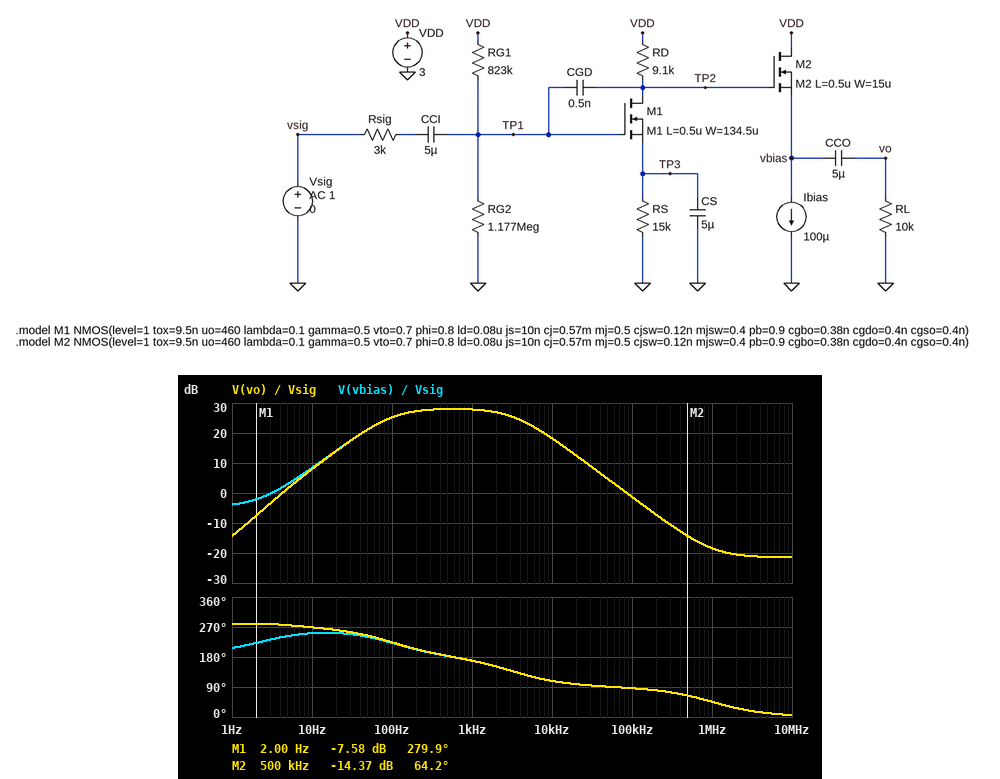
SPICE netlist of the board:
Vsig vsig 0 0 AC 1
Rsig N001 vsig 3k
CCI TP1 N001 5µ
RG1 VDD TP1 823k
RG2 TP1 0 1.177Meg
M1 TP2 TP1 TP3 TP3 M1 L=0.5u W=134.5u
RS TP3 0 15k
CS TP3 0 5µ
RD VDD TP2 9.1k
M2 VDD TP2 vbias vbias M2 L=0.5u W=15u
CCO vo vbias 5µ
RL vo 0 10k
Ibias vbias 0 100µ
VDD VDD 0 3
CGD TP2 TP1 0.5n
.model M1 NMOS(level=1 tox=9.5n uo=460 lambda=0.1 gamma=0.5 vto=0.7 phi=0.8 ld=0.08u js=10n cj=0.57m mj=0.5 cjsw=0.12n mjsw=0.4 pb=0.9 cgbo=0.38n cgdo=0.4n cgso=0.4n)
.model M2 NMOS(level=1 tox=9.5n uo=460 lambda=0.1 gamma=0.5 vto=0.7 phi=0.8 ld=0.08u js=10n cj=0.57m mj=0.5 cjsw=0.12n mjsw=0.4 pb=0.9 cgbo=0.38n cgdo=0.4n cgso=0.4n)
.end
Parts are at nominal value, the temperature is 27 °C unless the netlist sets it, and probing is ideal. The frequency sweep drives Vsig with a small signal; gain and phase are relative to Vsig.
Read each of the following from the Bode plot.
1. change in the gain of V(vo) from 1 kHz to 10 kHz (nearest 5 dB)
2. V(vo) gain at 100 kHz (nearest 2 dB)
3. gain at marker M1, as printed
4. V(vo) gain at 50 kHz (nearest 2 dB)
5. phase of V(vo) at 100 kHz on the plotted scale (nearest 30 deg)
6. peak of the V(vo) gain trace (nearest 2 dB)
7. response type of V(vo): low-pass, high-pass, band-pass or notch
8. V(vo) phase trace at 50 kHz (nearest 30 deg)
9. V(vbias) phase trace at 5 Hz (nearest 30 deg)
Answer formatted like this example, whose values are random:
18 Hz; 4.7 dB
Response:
-10 dB; -2 dB; -7.58 dB; 4 dB; 90 deg; 28 dB; band-pass; 90 deg; 240 deg
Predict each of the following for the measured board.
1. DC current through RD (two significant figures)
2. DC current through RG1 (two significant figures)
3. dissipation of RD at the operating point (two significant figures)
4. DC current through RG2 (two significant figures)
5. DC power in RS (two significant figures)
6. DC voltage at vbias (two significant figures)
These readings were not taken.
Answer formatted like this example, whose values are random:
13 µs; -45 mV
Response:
68 µA; 1.5 µA; 42 µW; 1.5 µA; 70 µW; 1.5 V
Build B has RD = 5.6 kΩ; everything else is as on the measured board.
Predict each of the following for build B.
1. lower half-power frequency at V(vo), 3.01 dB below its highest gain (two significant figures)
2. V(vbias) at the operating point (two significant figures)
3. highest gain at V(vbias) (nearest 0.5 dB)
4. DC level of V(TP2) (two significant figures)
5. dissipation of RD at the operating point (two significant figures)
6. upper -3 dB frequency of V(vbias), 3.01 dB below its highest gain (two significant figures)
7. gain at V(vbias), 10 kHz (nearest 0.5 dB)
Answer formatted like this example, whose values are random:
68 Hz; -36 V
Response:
100 Hz; 1.8 V; 24.0 dB; 2.6 V; 26 µW; 5.4 kHz; 17.5 dB
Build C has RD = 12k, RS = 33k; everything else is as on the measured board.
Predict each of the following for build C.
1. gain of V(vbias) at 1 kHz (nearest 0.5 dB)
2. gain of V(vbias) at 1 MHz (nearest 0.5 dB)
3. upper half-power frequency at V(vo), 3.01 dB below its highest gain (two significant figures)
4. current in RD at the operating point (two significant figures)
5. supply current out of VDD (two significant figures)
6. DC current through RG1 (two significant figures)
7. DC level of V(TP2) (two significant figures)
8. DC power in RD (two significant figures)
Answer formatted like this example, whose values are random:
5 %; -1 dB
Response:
27.0 dB; -17.0 dB; 3.6 kHz; 31 µA; 130 µA; 1.5 µA; 2.6 V; 12 µW
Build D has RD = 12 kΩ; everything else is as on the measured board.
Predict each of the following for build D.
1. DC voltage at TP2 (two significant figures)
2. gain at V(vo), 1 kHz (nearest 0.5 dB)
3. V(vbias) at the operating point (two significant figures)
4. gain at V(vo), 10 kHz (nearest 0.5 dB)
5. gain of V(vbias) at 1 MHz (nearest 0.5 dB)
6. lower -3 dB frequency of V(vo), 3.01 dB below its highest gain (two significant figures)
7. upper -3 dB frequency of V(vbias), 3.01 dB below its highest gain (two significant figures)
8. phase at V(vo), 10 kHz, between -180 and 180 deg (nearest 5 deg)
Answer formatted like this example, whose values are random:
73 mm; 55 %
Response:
2.2 V; 30.0 dB; 1.3 V; 18.5 dB; -18.5 dB; 92 Hz; 2.8 kHz; 105 deg
